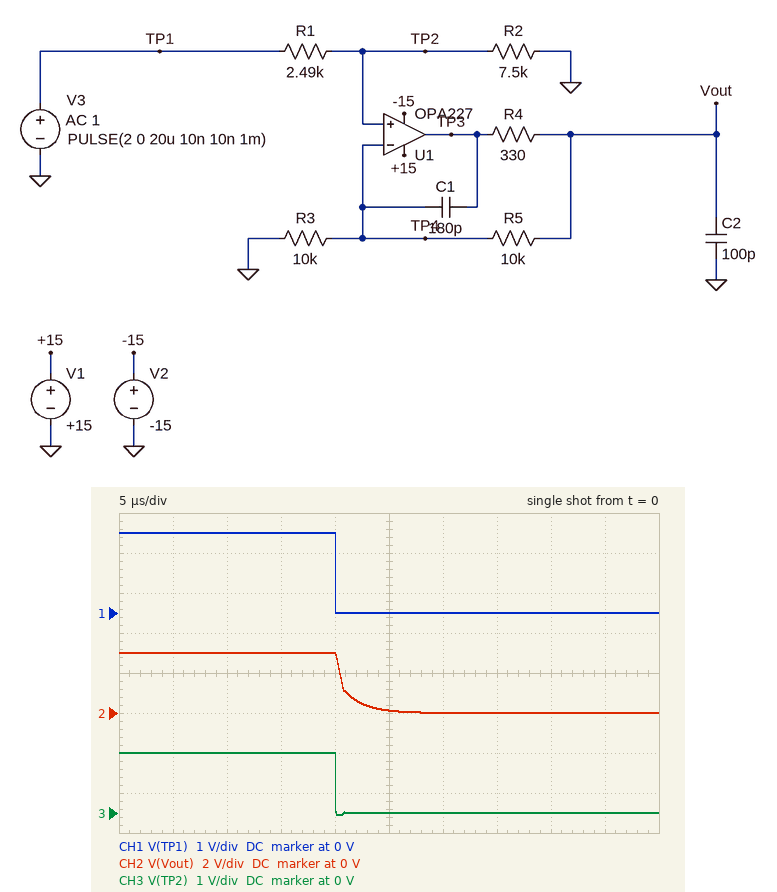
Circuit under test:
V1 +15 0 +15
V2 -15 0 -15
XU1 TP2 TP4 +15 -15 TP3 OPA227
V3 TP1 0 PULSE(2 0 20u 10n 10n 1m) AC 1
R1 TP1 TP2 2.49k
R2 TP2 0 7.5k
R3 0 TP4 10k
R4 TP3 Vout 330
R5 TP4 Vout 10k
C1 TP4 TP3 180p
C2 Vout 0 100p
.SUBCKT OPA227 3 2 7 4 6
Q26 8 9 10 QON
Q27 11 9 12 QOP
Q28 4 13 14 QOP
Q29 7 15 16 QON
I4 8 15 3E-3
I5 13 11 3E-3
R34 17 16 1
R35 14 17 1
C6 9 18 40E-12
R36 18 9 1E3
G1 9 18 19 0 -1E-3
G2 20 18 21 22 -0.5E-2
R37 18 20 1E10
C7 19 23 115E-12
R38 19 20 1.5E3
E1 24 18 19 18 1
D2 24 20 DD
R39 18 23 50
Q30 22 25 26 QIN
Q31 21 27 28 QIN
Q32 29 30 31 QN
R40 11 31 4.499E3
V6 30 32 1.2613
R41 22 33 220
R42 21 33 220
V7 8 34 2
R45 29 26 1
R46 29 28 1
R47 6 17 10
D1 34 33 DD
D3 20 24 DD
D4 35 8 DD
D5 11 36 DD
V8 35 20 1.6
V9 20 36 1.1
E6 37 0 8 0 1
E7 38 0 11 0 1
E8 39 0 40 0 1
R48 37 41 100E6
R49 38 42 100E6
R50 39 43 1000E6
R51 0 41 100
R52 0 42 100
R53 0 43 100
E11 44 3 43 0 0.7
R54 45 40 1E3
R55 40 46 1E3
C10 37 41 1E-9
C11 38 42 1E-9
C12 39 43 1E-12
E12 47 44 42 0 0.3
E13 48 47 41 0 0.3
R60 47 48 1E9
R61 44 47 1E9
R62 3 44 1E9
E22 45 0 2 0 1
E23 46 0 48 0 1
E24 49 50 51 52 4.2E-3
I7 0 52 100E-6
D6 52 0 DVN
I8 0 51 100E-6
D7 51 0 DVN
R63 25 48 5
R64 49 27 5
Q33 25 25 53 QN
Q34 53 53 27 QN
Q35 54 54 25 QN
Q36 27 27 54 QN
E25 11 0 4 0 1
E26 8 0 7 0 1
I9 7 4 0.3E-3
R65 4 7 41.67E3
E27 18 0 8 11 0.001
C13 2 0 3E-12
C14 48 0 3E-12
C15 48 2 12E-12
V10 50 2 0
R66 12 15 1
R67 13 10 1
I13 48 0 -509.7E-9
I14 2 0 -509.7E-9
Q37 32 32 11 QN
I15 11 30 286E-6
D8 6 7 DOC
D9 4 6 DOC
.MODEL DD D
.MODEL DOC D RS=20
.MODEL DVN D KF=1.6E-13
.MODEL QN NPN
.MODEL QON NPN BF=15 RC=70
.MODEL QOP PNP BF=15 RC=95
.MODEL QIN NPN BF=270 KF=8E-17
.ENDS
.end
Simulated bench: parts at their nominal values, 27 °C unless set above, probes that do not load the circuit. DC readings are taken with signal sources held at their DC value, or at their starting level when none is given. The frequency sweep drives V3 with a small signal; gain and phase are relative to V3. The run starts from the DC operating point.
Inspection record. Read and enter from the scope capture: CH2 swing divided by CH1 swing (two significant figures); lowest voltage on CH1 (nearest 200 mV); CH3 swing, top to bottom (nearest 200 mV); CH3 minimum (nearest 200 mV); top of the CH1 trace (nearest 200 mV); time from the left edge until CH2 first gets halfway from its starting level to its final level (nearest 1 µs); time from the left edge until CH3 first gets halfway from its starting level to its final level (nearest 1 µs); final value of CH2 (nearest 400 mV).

1.5
0 V
1.6 V
0 V
2.0 V
21 µs
20 µs
0 V
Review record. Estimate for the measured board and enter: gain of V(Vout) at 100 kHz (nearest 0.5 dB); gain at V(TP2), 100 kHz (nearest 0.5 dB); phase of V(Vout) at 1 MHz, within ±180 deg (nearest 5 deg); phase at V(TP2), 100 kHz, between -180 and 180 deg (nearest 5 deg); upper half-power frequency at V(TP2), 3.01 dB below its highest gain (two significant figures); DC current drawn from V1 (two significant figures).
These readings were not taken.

1.0 dB
-2.5 dB
-25 deg
0 deg
5.3 MHz
3.7 mA
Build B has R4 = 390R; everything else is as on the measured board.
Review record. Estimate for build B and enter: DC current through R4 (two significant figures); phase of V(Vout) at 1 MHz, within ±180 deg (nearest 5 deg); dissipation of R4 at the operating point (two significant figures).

150 µA
-30 deg
8.8 µW
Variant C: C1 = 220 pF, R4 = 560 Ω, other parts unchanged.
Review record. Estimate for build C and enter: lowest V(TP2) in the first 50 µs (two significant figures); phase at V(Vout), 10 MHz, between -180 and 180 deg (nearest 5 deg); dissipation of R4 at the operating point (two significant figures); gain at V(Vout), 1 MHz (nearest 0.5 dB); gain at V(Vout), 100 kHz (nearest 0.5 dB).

-48 mV
90 deg
13 µW
-2.5 dB
0.5 dB
